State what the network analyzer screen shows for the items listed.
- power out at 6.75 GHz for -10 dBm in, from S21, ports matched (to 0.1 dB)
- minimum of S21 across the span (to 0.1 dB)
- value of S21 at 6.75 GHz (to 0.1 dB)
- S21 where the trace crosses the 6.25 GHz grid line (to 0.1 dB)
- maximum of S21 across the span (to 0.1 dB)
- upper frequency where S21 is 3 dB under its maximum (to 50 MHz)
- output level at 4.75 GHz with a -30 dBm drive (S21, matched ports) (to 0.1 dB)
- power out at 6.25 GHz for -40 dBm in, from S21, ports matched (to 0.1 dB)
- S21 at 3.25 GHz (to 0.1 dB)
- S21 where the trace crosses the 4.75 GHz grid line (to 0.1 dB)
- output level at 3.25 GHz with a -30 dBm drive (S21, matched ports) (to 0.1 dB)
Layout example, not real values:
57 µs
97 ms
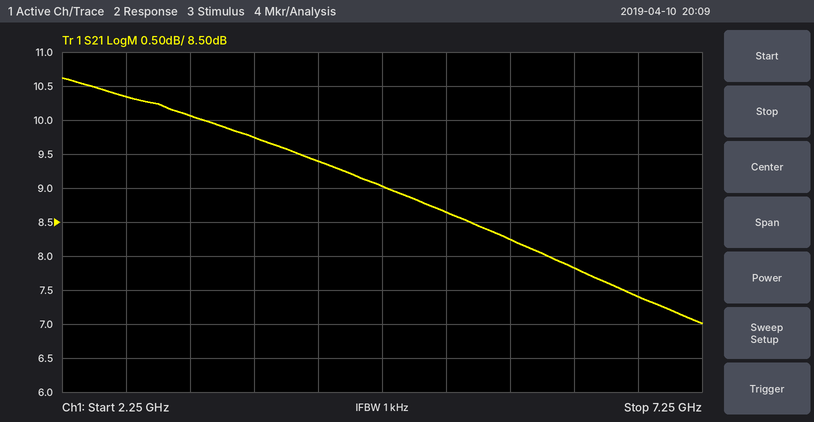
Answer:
-2.6 dBm
7.0 dB
7.4 dB
7.8 dB
10.6 dB
6.50 GHz
-21.0 dBm
-32.2 dBm
10.1 dB
9.0 dB
-19.9 dBm
